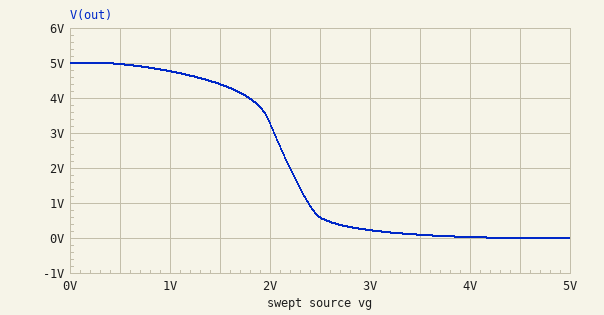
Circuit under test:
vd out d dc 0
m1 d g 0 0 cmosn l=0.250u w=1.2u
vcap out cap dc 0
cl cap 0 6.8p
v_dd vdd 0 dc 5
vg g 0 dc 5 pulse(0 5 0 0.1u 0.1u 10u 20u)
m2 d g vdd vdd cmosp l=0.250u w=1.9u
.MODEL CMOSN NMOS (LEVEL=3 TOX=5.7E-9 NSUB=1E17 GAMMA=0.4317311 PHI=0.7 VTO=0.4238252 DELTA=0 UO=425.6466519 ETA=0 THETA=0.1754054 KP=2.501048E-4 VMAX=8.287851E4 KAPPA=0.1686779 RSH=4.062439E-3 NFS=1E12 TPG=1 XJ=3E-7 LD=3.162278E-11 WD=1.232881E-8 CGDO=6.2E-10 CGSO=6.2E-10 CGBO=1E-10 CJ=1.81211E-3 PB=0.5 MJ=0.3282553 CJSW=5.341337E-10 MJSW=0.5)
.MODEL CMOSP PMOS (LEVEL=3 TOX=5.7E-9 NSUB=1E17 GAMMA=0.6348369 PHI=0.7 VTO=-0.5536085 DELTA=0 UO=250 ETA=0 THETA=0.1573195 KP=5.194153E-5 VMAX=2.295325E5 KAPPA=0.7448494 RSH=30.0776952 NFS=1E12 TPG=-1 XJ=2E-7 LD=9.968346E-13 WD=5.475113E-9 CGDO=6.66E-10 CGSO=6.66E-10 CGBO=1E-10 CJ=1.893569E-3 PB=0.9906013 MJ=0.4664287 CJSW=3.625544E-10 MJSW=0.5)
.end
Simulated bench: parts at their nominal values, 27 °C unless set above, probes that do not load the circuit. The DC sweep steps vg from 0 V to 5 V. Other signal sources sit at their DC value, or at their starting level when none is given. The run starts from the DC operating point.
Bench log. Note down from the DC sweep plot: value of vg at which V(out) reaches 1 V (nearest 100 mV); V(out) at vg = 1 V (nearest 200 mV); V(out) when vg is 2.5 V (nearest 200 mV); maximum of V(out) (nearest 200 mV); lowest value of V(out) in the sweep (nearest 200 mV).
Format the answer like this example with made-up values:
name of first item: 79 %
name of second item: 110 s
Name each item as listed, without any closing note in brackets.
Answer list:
value of vg at which V(out) reaches 1 V: 2.4 V
V(out) at vg = 1 V: 4.8 V
V(out) when vg is 2.5 V: 600 mV
maximum of V(out): 5.0 V
lowest value of V(out) in the sweep: 0 V
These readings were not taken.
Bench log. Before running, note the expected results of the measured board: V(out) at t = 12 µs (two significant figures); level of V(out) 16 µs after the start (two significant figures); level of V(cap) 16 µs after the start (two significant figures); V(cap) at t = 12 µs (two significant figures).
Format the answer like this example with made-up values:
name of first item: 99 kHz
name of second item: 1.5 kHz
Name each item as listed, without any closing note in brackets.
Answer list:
V(out) at t = 12 µs: 5.0 V
level of V(out) 16 µs after the start: 5.0 V
level of V(cap) 16 µs after the start: 5.0 V
V(cap) at t = 12 µs: 5.0 V
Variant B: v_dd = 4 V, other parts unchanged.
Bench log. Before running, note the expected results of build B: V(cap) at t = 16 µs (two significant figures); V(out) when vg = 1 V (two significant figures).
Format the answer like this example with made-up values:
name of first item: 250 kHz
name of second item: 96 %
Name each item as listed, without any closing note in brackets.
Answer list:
V(cap) at t = 16 µs: 4.0 V
V(out) when vg = 1 V: 3.7 V
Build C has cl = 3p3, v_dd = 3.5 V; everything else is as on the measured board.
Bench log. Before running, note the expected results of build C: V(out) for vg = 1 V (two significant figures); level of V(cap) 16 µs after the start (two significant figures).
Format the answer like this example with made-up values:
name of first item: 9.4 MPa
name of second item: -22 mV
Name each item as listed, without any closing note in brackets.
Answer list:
V(out) for vg = 1 V: 3.2 V
level of V(cap) 16 µs after the start: 3.5 V
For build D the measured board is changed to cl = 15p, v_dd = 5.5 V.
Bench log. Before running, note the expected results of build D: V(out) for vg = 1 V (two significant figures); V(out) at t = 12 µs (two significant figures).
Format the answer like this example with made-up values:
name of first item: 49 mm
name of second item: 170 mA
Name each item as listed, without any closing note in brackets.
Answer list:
V(out) for vg = 1 V: 5.3 V
V(out) at t = 12 µs: 5.5 V
